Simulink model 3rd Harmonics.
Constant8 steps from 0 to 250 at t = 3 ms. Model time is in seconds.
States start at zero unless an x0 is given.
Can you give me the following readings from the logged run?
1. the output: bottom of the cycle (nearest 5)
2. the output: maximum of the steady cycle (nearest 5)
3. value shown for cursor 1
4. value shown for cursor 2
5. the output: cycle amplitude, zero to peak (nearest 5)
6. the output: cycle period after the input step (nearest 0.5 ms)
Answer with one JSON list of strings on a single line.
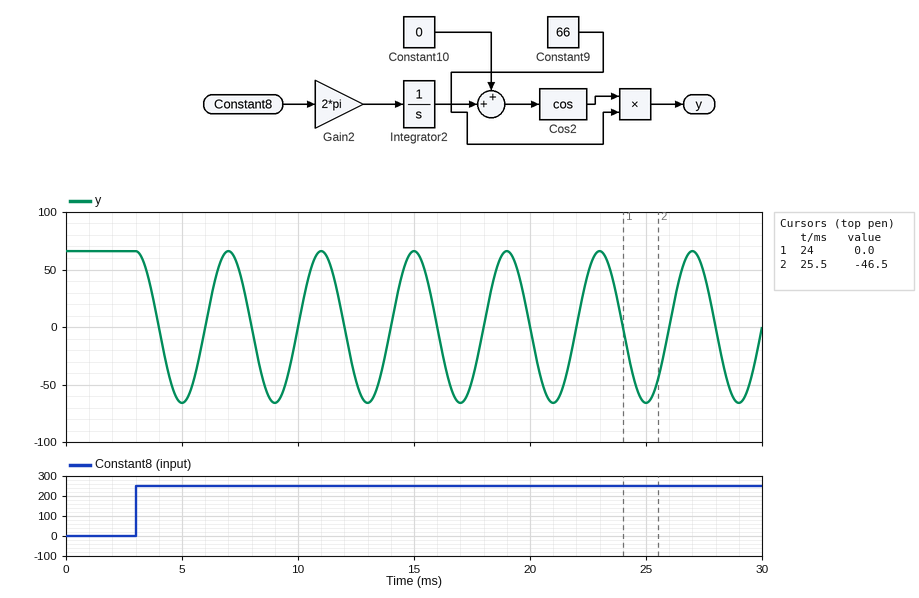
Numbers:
["-65", "65", "0.0", "-46.5", "65", "4.0 ms"]
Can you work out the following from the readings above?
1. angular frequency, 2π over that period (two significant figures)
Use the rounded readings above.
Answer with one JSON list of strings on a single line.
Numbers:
["1.6 rad/ms"]
